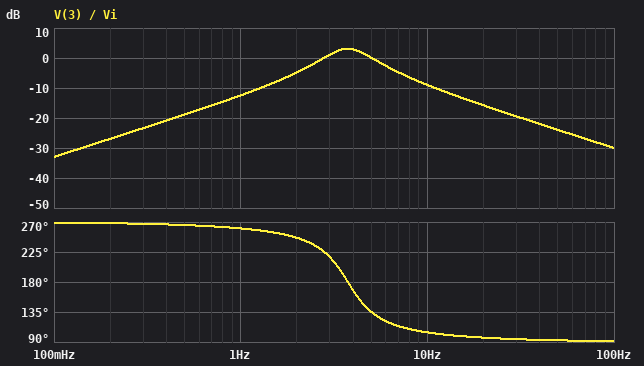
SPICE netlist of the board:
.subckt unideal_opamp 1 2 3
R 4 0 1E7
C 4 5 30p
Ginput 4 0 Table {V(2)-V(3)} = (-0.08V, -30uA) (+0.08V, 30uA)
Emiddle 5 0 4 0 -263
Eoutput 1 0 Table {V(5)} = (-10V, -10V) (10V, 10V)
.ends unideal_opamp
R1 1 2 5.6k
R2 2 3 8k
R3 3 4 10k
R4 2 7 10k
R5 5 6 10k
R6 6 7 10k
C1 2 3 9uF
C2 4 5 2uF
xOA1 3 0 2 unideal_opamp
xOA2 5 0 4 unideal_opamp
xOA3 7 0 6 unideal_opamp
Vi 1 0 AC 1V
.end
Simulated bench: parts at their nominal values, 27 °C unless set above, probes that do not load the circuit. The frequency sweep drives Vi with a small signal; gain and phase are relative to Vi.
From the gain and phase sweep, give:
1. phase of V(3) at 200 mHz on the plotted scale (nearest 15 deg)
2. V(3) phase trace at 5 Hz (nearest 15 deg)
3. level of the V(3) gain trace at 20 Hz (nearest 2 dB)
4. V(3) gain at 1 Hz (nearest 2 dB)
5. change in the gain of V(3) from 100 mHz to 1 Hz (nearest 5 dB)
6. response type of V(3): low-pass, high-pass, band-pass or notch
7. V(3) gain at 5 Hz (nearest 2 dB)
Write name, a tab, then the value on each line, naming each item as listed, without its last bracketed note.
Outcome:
phase of V(3) at 200 mHz on the plotted scale	270 deg
V(3) phase trace at 5 Hz	135 deg
level of the V(3) gain trace at 20 Hz	-16 dB
V(3) gain at 1 Hz	-12 dB
change in the gain of V(3) from 100 mHz to 1 Hz	20 dB
response type of V(3): low-pass, high-pass, band-pass or notch	band-pass
V(3) gain at 5 Hz	0 dB
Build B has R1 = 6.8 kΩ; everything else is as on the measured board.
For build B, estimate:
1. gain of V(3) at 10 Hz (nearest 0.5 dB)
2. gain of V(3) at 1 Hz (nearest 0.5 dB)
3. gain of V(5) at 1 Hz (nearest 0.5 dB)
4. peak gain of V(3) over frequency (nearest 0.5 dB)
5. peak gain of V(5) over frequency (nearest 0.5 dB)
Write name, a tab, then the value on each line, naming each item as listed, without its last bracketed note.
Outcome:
gain of V(3) at 10 Hz	-10.5 dB
gain of V(3) at 1 Hz	-14.0 dB
gain of V(5) at 1 Hz	4.0 dB
peak gain of V(3) over frequency	1.5 dB
peak gain of V(5) over frequency	8.5 dB
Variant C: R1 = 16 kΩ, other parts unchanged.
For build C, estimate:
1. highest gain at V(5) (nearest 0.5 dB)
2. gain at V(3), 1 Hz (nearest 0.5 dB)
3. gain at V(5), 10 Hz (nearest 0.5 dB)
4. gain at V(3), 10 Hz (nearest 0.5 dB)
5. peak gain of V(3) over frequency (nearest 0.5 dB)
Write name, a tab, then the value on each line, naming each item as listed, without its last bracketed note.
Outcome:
highest gain at V(5)	1.0 dB
gain at V(3), 1 Hz	-21.5 dB
gain at V(5), 10 Hz	-20.0 dB
gain at V(3), 10 Hz	-18.0 dB
peak gain of V(3) over frequency	-6.0 dB
